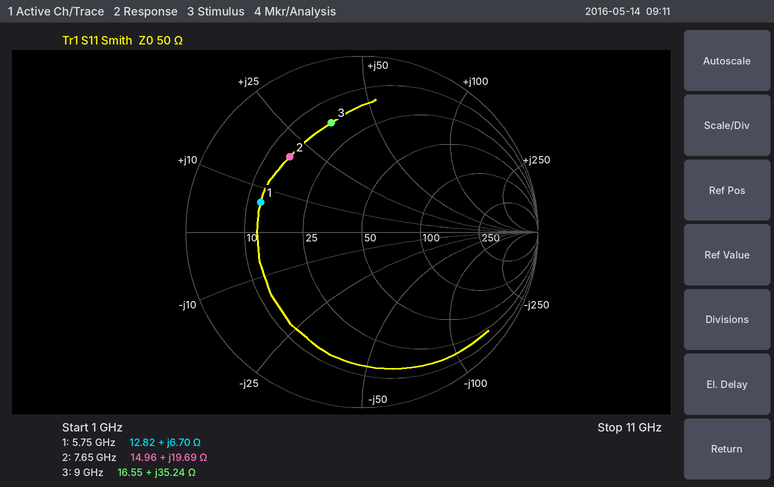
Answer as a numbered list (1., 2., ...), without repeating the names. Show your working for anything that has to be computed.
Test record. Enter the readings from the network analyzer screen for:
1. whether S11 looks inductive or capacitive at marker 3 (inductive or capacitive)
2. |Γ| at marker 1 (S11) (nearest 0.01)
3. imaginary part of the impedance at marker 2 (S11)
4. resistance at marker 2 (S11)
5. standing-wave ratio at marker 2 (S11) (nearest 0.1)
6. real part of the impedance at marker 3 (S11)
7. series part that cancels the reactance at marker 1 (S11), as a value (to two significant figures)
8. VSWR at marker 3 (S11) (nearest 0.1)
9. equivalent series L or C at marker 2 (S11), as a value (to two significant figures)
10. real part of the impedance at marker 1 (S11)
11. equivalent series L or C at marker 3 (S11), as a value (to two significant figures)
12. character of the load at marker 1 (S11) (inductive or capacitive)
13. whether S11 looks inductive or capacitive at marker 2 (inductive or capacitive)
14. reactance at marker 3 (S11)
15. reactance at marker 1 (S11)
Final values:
1. inductive
2. 0.60
3. +19.69 Ω
4. 14.96 Ω
5. 3.9
6. 16.55 Ω
7. C = 1/(2π × 5.75 GHz × 6.7 Ω) ≈ 4.1 pF
8. 4.6
9. L = 19.69 Ω/(2π × 7.65 GHz) ≈ 410 pH
10. 12.82 Ω
11. L = 35.24 Ω/(2π × 9 GHz) ≈ 623 pH, so 620 pH to two significant figures
12. inductive
13. inductive
14. +35.24 Ω
15. +6.70 Ω
